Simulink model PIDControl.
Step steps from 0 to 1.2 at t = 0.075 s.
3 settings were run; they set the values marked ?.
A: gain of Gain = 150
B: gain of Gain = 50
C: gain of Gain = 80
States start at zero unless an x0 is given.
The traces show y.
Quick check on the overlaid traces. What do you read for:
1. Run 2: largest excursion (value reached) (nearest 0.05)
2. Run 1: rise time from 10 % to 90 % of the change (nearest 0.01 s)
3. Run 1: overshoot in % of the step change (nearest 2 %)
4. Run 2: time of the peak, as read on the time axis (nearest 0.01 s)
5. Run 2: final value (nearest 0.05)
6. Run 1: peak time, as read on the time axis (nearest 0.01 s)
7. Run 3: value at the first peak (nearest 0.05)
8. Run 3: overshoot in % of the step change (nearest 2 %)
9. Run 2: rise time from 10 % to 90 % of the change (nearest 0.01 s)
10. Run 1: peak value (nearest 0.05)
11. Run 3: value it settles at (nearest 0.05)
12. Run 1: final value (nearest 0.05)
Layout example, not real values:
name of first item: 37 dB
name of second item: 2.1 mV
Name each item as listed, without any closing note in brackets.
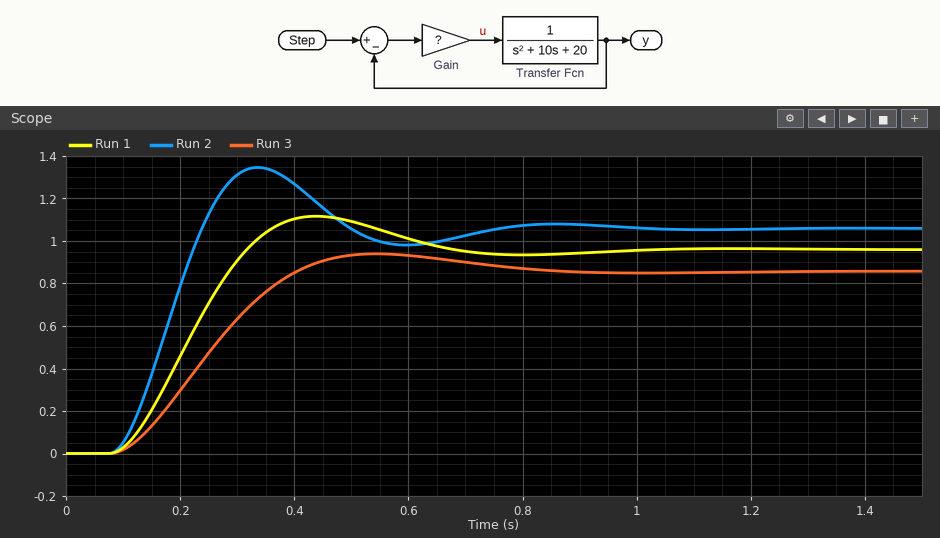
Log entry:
Run 2: largest excursion (value reached): 1.35
Run 1: rise time from 10 % to 90 % of the change: 0.16 s
Run 1: overshoot in % of the step change: 16 %
Run 2: time of the peak, as read on the time axis: 0.34 s
Run 2: final value: 1.05
Run 1: peak time, as read on the time axis: 0.44 s
Run 3: value at the first peak: 0.95
Run 3: overshoot in % of the step change: 10 %
Run 2: rise time from 10 % to 90 % of the change: 0.11 s
Run 1: peak value: 1.10
Run 3: value it settles at: 0.85
Run 1: final value: 0.95
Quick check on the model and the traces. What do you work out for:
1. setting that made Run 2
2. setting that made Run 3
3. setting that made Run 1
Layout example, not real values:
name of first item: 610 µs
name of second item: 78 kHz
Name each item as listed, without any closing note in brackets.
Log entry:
setting that made Run 2: A
setting that made Run 3: B
setting that made Run 1: C
